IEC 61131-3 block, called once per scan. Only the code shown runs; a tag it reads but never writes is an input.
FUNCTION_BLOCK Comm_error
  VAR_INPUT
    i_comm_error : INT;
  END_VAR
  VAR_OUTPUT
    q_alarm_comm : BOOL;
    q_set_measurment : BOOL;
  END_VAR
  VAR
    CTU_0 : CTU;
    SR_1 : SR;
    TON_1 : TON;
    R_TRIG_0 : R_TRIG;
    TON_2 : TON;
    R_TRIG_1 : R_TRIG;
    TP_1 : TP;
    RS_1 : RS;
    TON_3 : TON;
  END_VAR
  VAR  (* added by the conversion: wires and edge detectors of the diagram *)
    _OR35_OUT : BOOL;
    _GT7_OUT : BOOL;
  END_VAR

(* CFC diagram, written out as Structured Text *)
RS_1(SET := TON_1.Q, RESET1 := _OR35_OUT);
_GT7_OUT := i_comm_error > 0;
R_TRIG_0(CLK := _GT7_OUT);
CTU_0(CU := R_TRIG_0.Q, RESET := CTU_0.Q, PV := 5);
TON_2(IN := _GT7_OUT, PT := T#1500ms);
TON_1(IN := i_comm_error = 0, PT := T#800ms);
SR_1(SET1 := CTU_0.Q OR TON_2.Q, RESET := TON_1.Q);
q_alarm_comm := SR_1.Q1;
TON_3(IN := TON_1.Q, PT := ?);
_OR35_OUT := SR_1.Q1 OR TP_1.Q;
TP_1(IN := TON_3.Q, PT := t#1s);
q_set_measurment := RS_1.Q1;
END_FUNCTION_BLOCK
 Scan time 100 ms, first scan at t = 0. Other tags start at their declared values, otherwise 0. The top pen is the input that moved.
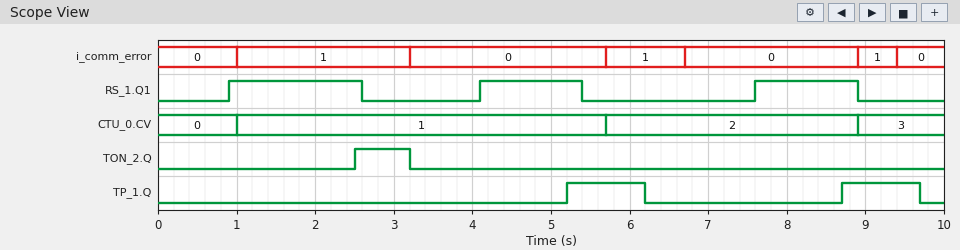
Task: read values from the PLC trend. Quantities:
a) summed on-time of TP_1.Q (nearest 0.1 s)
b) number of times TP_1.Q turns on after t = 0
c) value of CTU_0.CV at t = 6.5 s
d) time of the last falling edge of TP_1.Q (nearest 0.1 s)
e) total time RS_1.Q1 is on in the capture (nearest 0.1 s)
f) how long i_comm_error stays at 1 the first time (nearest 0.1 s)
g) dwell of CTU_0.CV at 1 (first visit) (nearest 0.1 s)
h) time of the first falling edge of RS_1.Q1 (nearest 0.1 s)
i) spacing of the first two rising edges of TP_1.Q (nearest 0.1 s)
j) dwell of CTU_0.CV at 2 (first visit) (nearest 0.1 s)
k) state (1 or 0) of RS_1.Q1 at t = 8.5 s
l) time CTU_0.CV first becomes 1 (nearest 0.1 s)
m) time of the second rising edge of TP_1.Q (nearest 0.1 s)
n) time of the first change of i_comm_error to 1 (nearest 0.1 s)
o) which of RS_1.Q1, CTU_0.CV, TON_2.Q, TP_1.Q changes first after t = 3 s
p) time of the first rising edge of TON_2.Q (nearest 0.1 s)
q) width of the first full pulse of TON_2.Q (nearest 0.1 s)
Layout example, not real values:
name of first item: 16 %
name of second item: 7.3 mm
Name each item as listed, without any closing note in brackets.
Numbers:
summed on-time of TP_1.Q: 2.0 s
number of times TP_1.Q turns on after t = 0: 2
value of CTU_0.CV at t = 6.5 s: 2
time of the last falling edge of TP_1.Q: 9.7 s
total time RS_1.Q1 is on in the capture: 4.3 s
how long i_comm_error stays at 1 the first time: 2.2 s
dwell of CTU_0.CV at 1 (first visit): 4.7 s
time of the first falling edge of RS_1.Q1: 2.6 s
spacing of the first two rising edges of TP_1.Q: 3.5 s
dwell of CTU_0.CV at 2 (first visit): 3.2 s
state (1 or 0) of RS_1.Q1 at t = 8.5 s: 1
time CTU_0.CV first becomes 1: 1.0 s
time of the second rising edge of TP_1.Q: 8.7 s
time of the first change of i_comm_error to 1: 1.0 s
which of RS_1.Q1, CTU_0.CV, TON_2.Q, TP_1.Q changes first after t = 3 s: TON_2.Q
time of the first rising edge of TON_2.Q: 2.5 s
width of the first full pulse of TON_2.Q: 0.7 s
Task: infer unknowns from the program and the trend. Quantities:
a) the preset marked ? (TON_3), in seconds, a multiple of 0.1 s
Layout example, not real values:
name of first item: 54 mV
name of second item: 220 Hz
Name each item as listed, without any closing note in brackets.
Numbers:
the preset marked ? (TON_3), in seconds, a multiple of 0.1 s: 1.2 s
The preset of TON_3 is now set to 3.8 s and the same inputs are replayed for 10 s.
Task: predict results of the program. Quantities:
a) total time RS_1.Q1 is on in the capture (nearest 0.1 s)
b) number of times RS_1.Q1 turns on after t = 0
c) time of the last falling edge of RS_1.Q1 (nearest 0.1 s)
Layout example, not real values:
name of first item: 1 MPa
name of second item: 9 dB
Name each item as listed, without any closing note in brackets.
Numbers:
total time RS_1.Q1 is on in the capture: 7.6 s
number of times RS_1.Q1 turns on after t = 0: 2
time of the last falling edge of RS_1.Q1: 2.6 s
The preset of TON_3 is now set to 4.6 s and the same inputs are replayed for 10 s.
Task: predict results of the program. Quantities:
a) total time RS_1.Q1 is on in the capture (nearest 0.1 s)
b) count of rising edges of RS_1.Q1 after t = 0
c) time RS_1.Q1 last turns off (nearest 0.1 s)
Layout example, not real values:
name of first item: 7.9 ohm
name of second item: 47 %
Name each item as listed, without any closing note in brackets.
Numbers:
total time RS_1.Q1 is on in the capture: 7.6 s
count of rising edges of RS_1.Q1 after t = 0: 2
time RS_1.Q1 last turns off: 2.6 s
